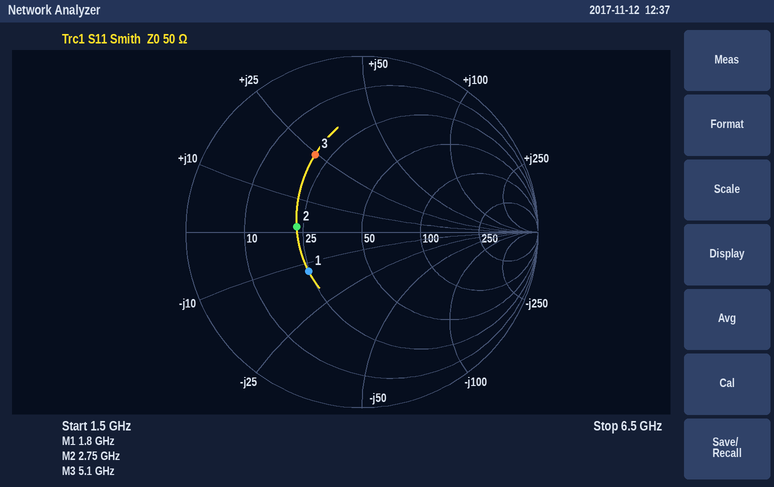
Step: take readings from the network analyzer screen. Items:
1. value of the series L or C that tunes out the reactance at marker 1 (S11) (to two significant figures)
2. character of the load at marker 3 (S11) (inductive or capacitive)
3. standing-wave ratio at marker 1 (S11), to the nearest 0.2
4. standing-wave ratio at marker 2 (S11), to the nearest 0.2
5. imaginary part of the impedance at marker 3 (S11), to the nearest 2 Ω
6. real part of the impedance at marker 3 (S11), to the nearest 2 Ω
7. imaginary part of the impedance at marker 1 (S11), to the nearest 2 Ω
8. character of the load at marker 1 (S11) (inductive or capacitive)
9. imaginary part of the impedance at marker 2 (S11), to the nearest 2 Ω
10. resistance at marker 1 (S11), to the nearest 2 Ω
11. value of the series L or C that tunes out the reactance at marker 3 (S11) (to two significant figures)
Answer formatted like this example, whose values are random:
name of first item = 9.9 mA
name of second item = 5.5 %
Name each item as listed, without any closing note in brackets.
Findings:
value of the series L or C that tunes out the reactance at marker 1 (S11) = 1.1 nH
character of the load at marker 3 (S11) = inductive
standing-wave ratio at marker 1 (S11), to the nearest 0.2 = 2.2
standing-wave ratio at marker 2 (S11), to the nearest 0.2 = 2.2
imaginary part of the impedance at marker 3 (S11), to the nearest 2 Ω = +24 Ω
real part of the impedance at marker 3 (S11), to the nearest 2 Ω = 20 Ω
imaginary part of the impedance at marker 1 (S11), to the nearest 2 Ω = -12 Ω
character of the load at marker 1 (S11) = capacitive
imaginary part of the impedance at marker 2 (S11), to the nearest 2 Ω = +2 Ω
resistance at marker 1 (S11), to the nearest 2 Ω = 24 Ω
value of the series L or C that tunes out the reactance at marker 3 (S11) = 1.3 pF
